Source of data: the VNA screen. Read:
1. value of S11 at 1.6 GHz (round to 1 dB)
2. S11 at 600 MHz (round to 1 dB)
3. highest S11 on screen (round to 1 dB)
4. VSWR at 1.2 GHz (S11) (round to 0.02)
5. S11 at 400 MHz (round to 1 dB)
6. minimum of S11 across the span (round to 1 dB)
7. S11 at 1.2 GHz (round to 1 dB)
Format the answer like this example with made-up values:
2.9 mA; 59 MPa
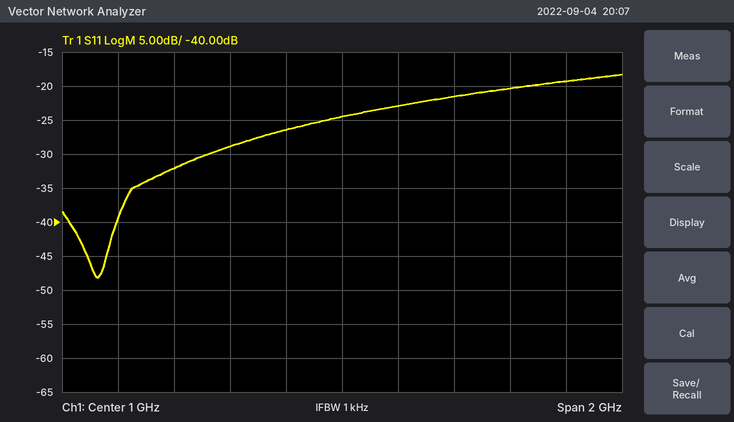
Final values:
-20 dB; -29 dB; -18 dB; 1.16; -32 dB; -48 dB; -23 dB
